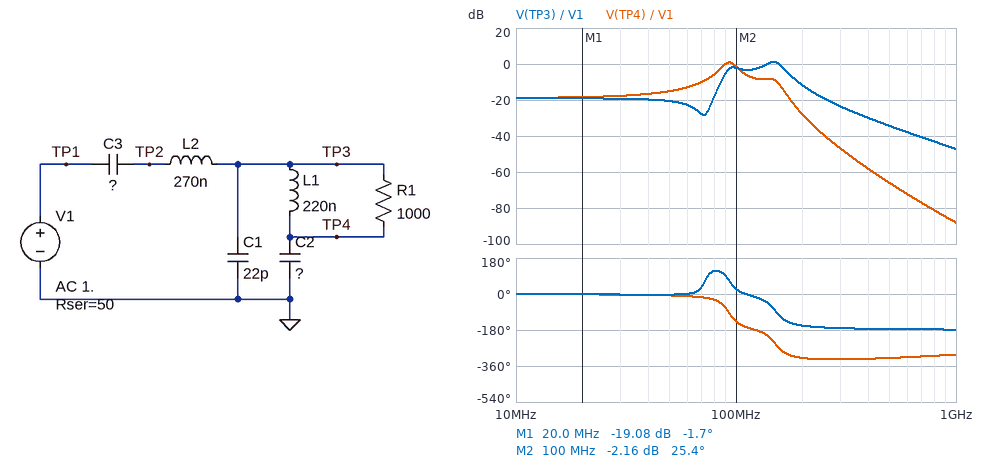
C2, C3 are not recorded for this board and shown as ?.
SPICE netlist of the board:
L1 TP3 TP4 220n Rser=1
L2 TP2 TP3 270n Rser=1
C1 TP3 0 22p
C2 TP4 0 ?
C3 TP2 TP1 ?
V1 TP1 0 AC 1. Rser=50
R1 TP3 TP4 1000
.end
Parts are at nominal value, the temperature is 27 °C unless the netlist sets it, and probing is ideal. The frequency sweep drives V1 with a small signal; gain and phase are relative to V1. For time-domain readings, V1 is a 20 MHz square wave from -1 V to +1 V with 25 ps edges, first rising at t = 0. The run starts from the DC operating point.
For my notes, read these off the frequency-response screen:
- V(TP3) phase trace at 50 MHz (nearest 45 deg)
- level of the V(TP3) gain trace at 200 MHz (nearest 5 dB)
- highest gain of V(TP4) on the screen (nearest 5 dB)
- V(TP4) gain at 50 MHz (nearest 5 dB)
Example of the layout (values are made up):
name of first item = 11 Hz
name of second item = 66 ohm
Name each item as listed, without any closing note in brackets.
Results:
V(TP3) phase trace at 50 MHz = 0 deg
level of the V(TP3) gain trace at 200 MHz = -10 dB
highest gain of V(TP4) on the screen = 0 dB
V(TP4) gain at 50 MHz = -15 dB
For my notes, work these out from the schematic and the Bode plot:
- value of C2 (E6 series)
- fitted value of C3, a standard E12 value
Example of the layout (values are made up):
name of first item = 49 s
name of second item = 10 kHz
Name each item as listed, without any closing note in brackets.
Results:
value of C2 = 22 pF
fitted value of C3, a standard E12 value = 5.6 pF
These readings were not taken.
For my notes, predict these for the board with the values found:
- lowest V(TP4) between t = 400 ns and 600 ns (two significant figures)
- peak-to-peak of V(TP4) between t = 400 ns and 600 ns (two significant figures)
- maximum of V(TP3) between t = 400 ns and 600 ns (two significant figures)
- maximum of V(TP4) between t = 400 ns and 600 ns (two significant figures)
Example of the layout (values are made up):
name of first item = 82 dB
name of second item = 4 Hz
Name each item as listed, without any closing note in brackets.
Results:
lowest V(TP4) between t = 400 ns and 600 ns = -370 mV
peak-to-peak of V(TP4) between t = 400 ns and 600 ns = 960 mV
maximum of V(TP3) between t = 400 ns and 600 ns = 600 mV
maximum of V(TP4) between t = 400 ns and 600 ns = 590 mV
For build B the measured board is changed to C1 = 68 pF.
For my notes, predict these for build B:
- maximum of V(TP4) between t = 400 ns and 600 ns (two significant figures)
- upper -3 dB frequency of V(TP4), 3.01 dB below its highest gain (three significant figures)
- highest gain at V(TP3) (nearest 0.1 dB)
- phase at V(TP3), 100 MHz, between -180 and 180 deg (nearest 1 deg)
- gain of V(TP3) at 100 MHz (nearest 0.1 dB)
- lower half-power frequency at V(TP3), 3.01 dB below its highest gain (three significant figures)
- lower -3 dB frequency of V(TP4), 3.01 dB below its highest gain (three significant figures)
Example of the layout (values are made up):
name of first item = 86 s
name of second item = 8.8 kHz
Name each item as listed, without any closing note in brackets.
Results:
maximum of V(TP4) between t = 400 ns and 600 ns = 250 mV
upper -3 dB frequency of V(TP4), 3.01 dB below its highest gain = 87.5 MHz
highest gain at V(TP3) = -8.3 dB
phase at V(TP3), 100 MHz, between -180 and 180 deg = -12 deg
gain of V(TP3) at 100 MHz = -13.2 dB
lower half-power frequency at V(TP3), 3.01 dB below its highest gain = 115 MHz
lower -3 dB frequency of V(TP4), 3.01 dB below its highest gain = 77.0 MHz
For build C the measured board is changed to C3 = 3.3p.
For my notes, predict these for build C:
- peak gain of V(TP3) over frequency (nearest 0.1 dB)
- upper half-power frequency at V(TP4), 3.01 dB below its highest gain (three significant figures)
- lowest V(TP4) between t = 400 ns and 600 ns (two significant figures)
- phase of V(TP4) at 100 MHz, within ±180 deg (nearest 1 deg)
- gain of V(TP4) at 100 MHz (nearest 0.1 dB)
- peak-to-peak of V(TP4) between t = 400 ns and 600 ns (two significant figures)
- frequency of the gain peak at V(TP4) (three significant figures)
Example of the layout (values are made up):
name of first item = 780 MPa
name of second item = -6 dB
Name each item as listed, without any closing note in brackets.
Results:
peak gain of V(TP3) over frequency = -1.0 dB
upper half-power frequency at V(TP4), 3.01 dB below its highest gain = 105 MHz
lowest V(TP4) between t = 400 ns and 600 ns = -250 mV
phase of V(TP4) at 100 MHz, within ±180 deg = -108 deg
gain of V(TP4) at 100 MHz = -4.2 dB
peak-to-peak of V(TP4) between t = 400 ns and 600 ns = 630 mV
frequency of the gain peak at V(TP4) = 97.4 MHz
